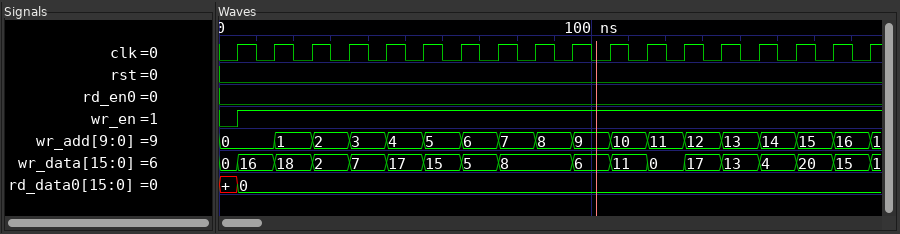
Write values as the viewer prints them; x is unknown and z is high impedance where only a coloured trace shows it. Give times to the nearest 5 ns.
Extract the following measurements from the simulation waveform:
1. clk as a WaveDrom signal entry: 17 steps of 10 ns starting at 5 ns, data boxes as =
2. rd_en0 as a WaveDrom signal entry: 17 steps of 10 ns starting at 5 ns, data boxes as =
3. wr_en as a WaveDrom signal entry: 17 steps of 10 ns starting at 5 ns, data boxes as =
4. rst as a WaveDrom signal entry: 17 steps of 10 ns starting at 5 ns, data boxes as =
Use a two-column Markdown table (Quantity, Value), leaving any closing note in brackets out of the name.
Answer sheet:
| Quantity | Value |
|---|---|
| clk as a WaveDrom signal entry: 17 steps of 10 ns starting at 5 ns, data boxes as = | {name: 'clk', wave: 'p................'} |
| rd_en0 as a WaveDrom signal entry: 17 steps of 10 ns starting at 5 ns, data boxes as = | {name: 'rd_en0', wave: '0................'} |
| wr_en as a WaveDrom signal entry: 17 steps of 10 ns starting at 5 ns, data boxes as = | {name: 'wr_en', wave: '1................'} |
| rst as a WaveDrom signal entry: 17 steps of 10 ns starting at 5 ns, data boxes as = | {name: 'rst', wave: '0................'} |
